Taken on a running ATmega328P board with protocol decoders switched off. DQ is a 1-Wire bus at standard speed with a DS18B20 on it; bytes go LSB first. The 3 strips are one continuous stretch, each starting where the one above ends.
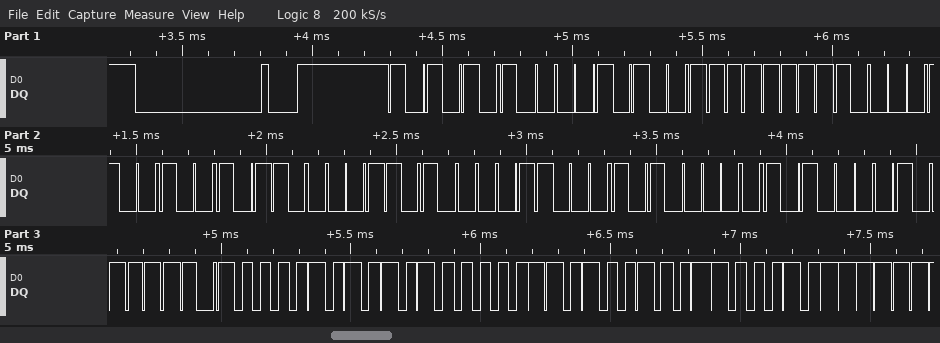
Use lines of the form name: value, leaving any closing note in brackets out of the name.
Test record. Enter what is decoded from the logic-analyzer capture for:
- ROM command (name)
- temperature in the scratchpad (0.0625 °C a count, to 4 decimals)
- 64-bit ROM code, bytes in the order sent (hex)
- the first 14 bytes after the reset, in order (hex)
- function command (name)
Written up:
ROM command: Match ROM
temperature in the scratchpad: 85.0000 °C
64-bit ROM code, bytes in the order sent: 28 FF 21 69 58 18 05 85
the first 14 bytes after the reset, in order: 55 28 FF 21 69 58 18 05 85 BE 50 05 4B 46
function command: Read Scratchpad
